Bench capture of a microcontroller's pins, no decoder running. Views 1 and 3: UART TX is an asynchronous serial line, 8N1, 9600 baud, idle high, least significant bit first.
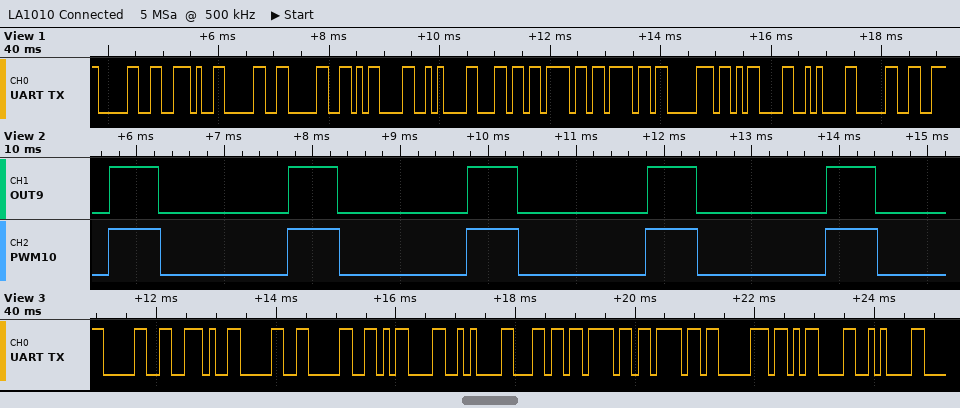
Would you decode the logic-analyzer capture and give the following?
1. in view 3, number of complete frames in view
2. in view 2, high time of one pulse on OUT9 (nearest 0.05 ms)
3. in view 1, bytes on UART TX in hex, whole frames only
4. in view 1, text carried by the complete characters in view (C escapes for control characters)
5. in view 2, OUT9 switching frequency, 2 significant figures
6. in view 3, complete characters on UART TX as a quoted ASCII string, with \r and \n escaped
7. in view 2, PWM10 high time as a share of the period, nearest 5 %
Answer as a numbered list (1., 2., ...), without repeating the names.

1. 12
2. 0.55 ms
3. 30 2E 30 30 0D 0A 6C 6F 6F 70 0D 0A 30
4. "0.00\r\nloop\r\n0"
5. 490 Hz
6. "0.00\r\nloop\r\n"
7. 30 %
